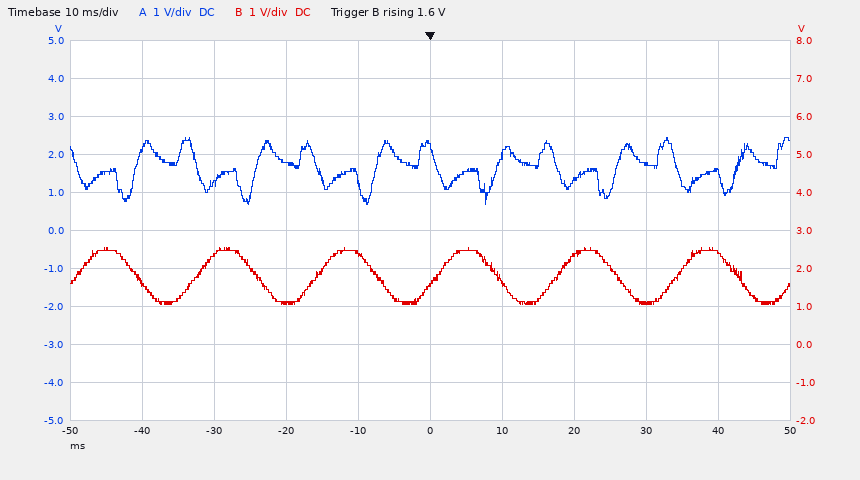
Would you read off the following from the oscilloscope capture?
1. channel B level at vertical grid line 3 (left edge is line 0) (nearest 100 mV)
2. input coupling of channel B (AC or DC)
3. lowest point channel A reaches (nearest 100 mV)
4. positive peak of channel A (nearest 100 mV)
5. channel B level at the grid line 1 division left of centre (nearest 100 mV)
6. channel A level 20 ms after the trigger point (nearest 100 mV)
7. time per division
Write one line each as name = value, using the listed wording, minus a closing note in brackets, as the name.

channel B level at vertical grid line 3 (left edge is line 0) = 1.1 V
input coupling of channel B = DC
lowest point channel A reaches = 700 mV
positive peak of channel A = 2.4 V
channel B level at the grid line 1 division left of centre = 2.4 V
channel A level 20 ms after the trigger point = 1.3 V
time per division = 10 ms
